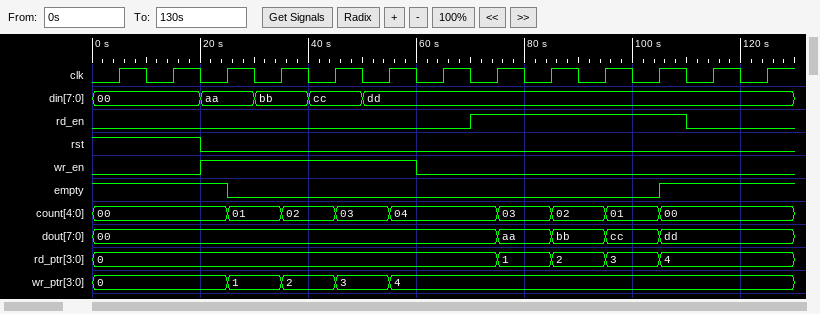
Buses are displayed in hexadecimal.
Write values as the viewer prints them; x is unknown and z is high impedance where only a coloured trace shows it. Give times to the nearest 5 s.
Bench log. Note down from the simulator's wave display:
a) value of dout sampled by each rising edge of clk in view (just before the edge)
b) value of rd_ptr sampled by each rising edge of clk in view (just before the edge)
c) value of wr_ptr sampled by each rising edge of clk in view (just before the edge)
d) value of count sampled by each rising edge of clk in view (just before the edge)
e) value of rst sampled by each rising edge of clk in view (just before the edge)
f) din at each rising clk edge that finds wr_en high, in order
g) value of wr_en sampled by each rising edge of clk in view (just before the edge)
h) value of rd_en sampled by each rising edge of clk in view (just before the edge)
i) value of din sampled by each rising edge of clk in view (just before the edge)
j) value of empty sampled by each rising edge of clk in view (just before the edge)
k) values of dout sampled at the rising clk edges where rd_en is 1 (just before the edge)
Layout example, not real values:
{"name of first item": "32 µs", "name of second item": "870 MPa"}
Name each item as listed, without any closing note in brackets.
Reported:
{"value of dout sampled by each rising edge of clk in view": "00, 00, 00, 00, 00, 00, 00, 00, aa, bb, cc, dd, dd", "value of rd_ptr sampled by each rising edge of clk in view": "0, 0, 0, 0, 0, 0, 0, 0, 1, 2, 3, 4, 4", "value of wr_ptr sampled by each rising edge of clk in view": "0, 0, 0, 1, 2, 3, 4, 4, 4, 4, 4, 4, 4", "value of count sampled by each rising edge of clk in view": "00, 00, 00, 01, 02, 03, 04, 04, 03, 02, 01, 00, 00", "value of rst sampled by each rising edge of clk in view": "1 1 0 0 0 0 0 0 0 0 0 0 0", "din at each rising clk edge that finds wr_en high, in order": "aa, bb, cc, dd", "value of wr_en sampled by each rising edge of clk in view": "0 0 1 1 1 1 0 0 0 0 0 0 0", "value of rd_en sampled by each rising edge of clk in view": "0 0 0 0 0 0 0 1 1 1 1 0 0", "value of din sampled by each rising edge of clk in view": "00, 00, aa, bb, cc, dd, dd, dd, dd, dd, dd, dd, dd", "value of empty sampled by each rising edge of clk in view": "1 1 1 0 0 0 0 0 0 0 0 1 1", "values of dout sampled at the rising clk edges where rd_en is 1": "00, aa, bb, cc"}
